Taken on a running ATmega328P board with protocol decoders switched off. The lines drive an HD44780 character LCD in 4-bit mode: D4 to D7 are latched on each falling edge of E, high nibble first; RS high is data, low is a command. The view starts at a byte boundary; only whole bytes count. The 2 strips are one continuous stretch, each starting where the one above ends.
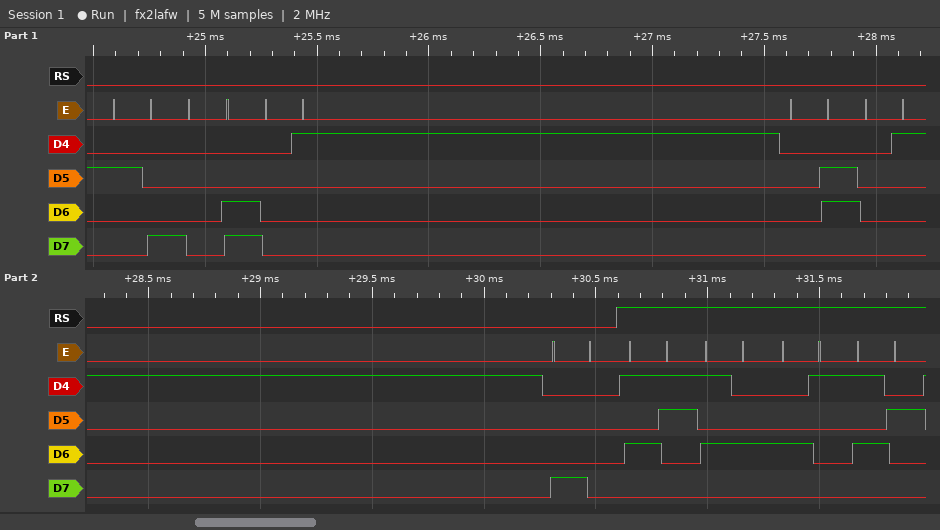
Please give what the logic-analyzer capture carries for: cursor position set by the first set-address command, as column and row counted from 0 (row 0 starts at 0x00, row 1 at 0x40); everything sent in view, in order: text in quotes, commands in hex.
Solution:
column 0, row 0
0x28 0x0C 0x01 0x06 0x01 0x80 "STAR"
